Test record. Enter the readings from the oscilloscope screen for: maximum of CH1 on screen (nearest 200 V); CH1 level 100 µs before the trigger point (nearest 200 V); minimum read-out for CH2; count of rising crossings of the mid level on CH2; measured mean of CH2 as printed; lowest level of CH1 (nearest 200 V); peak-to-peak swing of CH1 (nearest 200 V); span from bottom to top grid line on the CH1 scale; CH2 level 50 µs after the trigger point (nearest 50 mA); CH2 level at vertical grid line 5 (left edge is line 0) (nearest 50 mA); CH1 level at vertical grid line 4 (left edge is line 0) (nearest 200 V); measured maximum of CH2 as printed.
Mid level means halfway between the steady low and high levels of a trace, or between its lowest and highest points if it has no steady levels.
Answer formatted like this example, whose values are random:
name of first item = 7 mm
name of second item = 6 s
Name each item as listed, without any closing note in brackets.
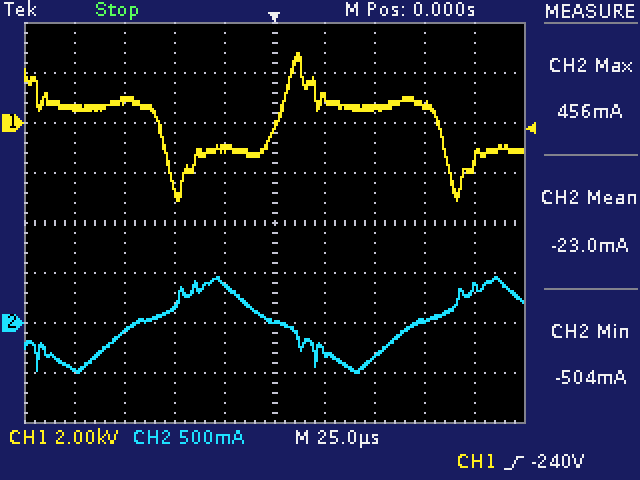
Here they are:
maximum of CH1 on screen = 2.8 kV
CH1 level 100 µs before the trigger point = 600 V
minimum read-out for CH2 = -504 mA
count of rising crossings of the mid level on CH2 = 2
measured mean of CH2 as printed = -23.0 mA
lowest level of CH1 = -3.2 kV
peak-to-peak swing of CH1 = 6.0 kV
span from bottom to top grid line on the CH1 scale = 16 kV
CH2 level 50 µs after the trigger point = -350 mA
CH2 level at vertical grid line 5 (left edge is line 0) = 0 mA
CH1 level at vertical grid line 4 (left edge is line 0) = -1.0 kV
measured maximum of CH2 as printed = 456 mA
